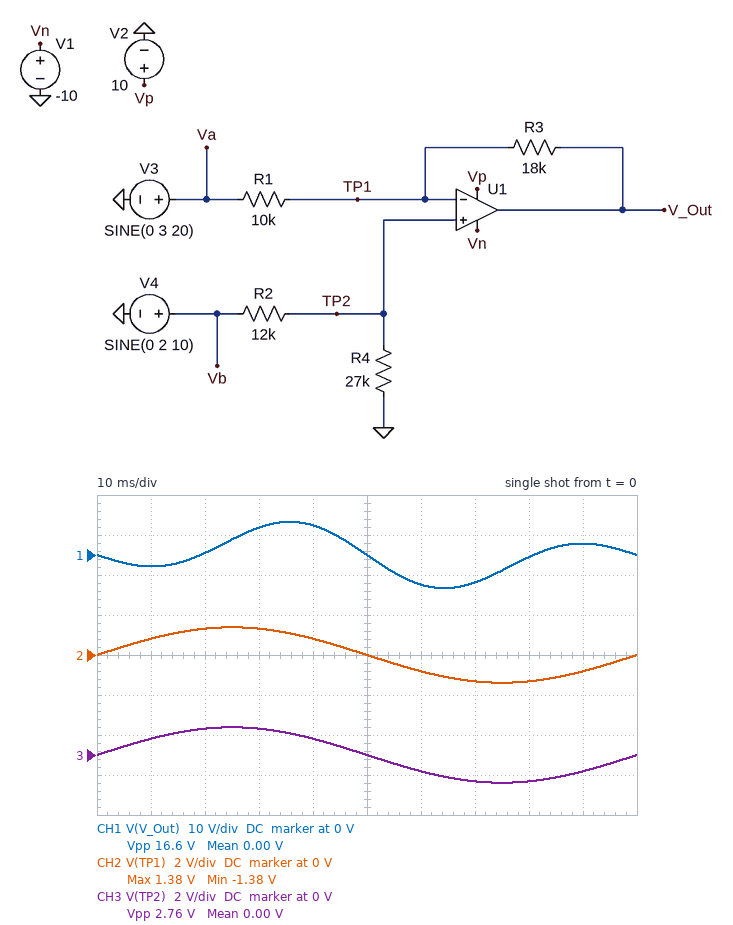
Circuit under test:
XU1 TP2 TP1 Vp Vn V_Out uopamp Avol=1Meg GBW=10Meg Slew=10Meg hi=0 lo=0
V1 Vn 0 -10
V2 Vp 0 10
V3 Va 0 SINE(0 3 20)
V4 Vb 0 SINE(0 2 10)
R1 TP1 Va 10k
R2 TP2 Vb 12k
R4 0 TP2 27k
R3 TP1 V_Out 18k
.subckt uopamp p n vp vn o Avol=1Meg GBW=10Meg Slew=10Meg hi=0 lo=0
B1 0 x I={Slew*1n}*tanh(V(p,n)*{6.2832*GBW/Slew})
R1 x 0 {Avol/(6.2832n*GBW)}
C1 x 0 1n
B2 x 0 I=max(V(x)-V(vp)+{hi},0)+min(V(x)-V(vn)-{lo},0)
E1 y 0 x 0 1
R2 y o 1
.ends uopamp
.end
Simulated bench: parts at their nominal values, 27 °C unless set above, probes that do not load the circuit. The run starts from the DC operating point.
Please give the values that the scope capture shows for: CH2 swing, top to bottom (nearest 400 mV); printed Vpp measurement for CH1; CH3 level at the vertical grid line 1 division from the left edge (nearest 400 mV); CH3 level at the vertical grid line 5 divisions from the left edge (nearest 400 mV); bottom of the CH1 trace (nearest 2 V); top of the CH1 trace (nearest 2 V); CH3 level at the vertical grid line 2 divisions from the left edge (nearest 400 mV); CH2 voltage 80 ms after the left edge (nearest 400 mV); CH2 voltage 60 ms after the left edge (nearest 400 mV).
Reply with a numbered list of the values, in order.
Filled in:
1. 2.8 V
2. 16.6 V
3. 800 mV
4. 0 V
5. -8 V
6. 8 V
7. 1.2 V
8. -1.2 V
9. -800 mV
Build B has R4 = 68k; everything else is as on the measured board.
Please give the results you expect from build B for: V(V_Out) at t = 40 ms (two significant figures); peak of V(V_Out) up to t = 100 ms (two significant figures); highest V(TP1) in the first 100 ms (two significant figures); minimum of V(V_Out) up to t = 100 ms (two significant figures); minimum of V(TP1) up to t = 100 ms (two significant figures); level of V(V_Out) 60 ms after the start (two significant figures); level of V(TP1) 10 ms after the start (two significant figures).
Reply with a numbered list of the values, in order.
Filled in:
1. 7.9 V
2. 9.0 V
3. 1.7 V
4. -9.0 V
5. -1.7 V
6. -7.9 V
7. 1.0 V
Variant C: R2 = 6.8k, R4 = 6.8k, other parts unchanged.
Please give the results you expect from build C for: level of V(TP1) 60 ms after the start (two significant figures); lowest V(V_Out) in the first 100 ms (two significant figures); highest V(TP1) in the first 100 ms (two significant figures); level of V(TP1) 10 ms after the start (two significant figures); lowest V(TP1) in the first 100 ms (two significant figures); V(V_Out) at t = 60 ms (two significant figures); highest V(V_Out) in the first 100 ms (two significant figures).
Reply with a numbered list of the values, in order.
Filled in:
1. -590 mV
2. -7.5 V
3. 1.0 V
4. 590 mV
5. -1.0 V
6. -6.8 V
7. 7.5 V
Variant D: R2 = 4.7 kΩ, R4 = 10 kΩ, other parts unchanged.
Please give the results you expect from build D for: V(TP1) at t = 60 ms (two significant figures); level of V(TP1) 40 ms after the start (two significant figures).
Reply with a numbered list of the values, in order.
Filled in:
1. -800 mV
2. 800 mV
